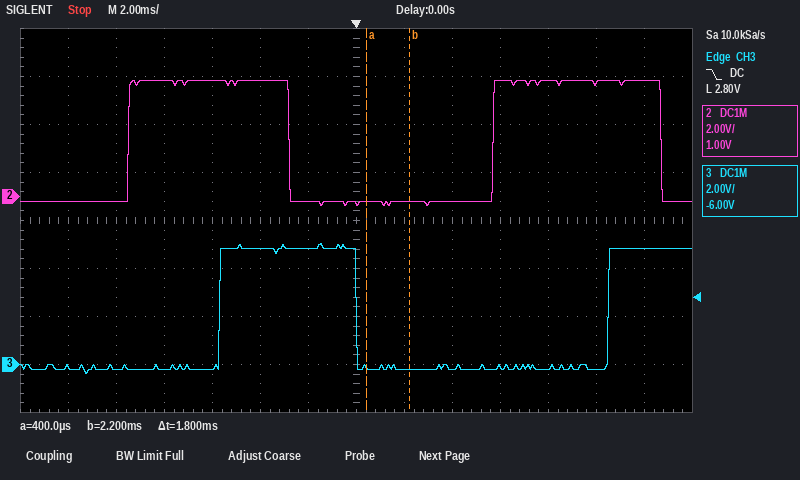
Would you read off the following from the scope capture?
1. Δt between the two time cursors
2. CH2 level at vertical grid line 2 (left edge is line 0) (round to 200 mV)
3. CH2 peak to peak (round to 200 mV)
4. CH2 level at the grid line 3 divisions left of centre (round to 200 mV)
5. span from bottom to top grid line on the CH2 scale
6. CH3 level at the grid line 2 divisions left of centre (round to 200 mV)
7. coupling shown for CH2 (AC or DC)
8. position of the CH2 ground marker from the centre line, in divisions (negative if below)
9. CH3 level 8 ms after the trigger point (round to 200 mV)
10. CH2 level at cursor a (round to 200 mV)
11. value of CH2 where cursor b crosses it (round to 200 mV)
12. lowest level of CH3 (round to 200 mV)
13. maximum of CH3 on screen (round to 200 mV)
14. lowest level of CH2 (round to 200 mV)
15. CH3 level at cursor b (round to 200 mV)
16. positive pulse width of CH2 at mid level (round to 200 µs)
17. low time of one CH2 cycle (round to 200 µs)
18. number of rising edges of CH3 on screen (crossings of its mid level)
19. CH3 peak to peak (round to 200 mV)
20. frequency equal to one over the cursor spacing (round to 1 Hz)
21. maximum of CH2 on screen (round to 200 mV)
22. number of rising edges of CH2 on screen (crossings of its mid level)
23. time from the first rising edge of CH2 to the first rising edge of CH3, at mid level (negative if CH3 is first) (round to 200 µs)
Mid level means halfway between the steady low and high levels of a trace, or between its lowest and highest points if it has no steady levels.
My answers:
1.8 ms
-200 mV
5.2 V
4.8 V
16 V
4.8 V
DC
+0.5 div
-200 mV
-200 mV
-200 mV
-400 mV
5.0 V
-400 mV
-200 mV
6.8 ms
8.4 ms
2
5.4 V
556 Hz
4.8 V
2
+3.8 ms
